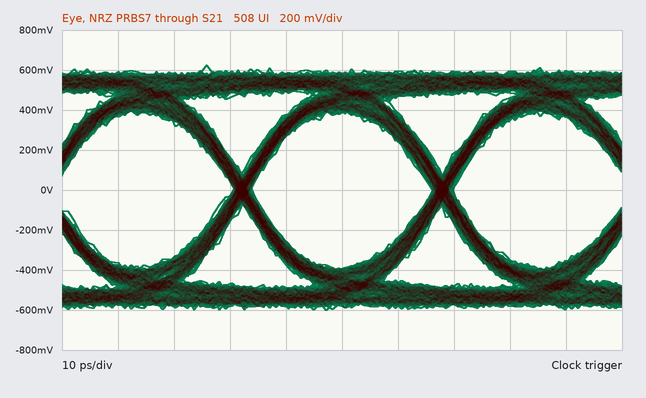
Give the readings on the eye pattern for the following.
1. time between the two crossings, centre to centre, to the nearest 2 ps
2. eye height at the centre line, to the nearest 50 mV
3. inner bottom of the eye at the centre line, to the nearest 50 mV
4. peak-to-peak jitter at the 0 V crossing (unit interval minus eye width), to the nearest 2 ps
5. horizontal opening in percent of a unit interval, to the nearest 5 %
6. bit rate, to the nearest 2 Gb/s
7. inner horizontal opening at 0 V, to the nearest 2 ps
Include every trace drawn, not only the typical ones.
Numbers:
36 ps
800 mV
-400 mV
4 ps
90 %
28 Gb/s
32 ps
